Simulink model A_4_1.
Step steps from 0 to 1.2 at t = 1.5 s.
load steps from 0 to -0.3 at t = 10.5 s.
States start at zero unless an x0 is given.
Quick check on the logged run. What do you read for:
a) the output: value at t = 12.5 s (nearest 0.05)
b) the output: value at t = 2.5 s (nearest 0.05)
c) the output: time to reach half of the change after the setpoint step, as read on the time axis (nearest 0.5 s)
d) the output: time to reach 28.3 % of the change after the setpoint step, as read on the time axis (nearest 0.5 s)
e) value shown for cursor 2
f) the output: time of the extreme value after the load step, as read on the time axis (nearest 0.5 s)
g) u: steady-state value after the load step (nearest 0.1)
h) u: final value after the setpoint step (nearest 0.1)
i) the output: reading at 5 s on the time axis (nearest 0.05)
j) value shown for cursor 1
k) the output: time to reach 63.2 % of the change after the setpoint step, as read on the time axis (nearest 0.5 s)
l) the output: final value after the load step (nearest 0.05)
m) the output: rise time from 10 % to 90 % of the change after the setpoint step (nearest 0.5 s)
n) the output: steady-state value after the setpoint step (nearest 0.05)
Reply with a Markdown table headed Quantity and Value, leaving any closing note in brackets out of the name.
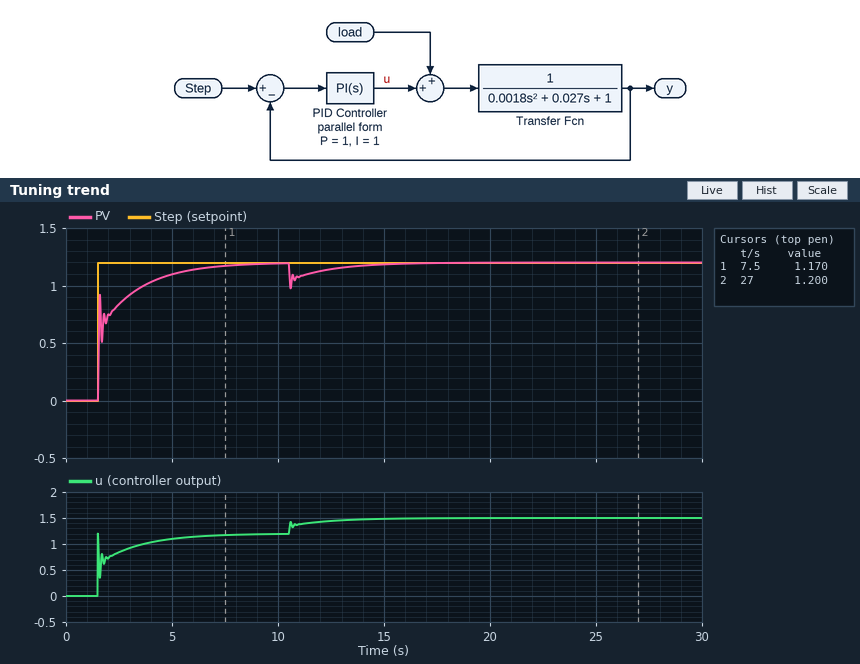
| Quantity | Value |
|---|---|
| the output: value at t = 12.5 s | 1.15 |
| the output: value at t = 2.5 s | 0.85 |
| the output: time to reach half of the change after the setpoint step, as read on the time axis | 1.5 s |
| the output: time to reach 28.3 % of the change after the setpoint step, as read on the time axis | 1.5 s |
| value shown for cursor 2 | 1.200 |
| the output: time of the extreme value after the load step, as read on the time axis | 10.5 s |
| u: steady-state value after the load step | 1.5 |
| u: final value after the setpoint step | 1.2 |
| the output: reading at 5 s on the time axis | 1.10 |
| value shown for cursor 1 | 1.170 |
| the output: time to reach 63.2 % of the change after the setpoint step, as read on the time axis | 1.5 s |
| the output: final value after the load step | 1.20 |
| the output: rise time from 10 % to 90 % of the change after the setpoint step | 3.0 s |
| the output: steady-state value after the setpoint step | 1.20 |
